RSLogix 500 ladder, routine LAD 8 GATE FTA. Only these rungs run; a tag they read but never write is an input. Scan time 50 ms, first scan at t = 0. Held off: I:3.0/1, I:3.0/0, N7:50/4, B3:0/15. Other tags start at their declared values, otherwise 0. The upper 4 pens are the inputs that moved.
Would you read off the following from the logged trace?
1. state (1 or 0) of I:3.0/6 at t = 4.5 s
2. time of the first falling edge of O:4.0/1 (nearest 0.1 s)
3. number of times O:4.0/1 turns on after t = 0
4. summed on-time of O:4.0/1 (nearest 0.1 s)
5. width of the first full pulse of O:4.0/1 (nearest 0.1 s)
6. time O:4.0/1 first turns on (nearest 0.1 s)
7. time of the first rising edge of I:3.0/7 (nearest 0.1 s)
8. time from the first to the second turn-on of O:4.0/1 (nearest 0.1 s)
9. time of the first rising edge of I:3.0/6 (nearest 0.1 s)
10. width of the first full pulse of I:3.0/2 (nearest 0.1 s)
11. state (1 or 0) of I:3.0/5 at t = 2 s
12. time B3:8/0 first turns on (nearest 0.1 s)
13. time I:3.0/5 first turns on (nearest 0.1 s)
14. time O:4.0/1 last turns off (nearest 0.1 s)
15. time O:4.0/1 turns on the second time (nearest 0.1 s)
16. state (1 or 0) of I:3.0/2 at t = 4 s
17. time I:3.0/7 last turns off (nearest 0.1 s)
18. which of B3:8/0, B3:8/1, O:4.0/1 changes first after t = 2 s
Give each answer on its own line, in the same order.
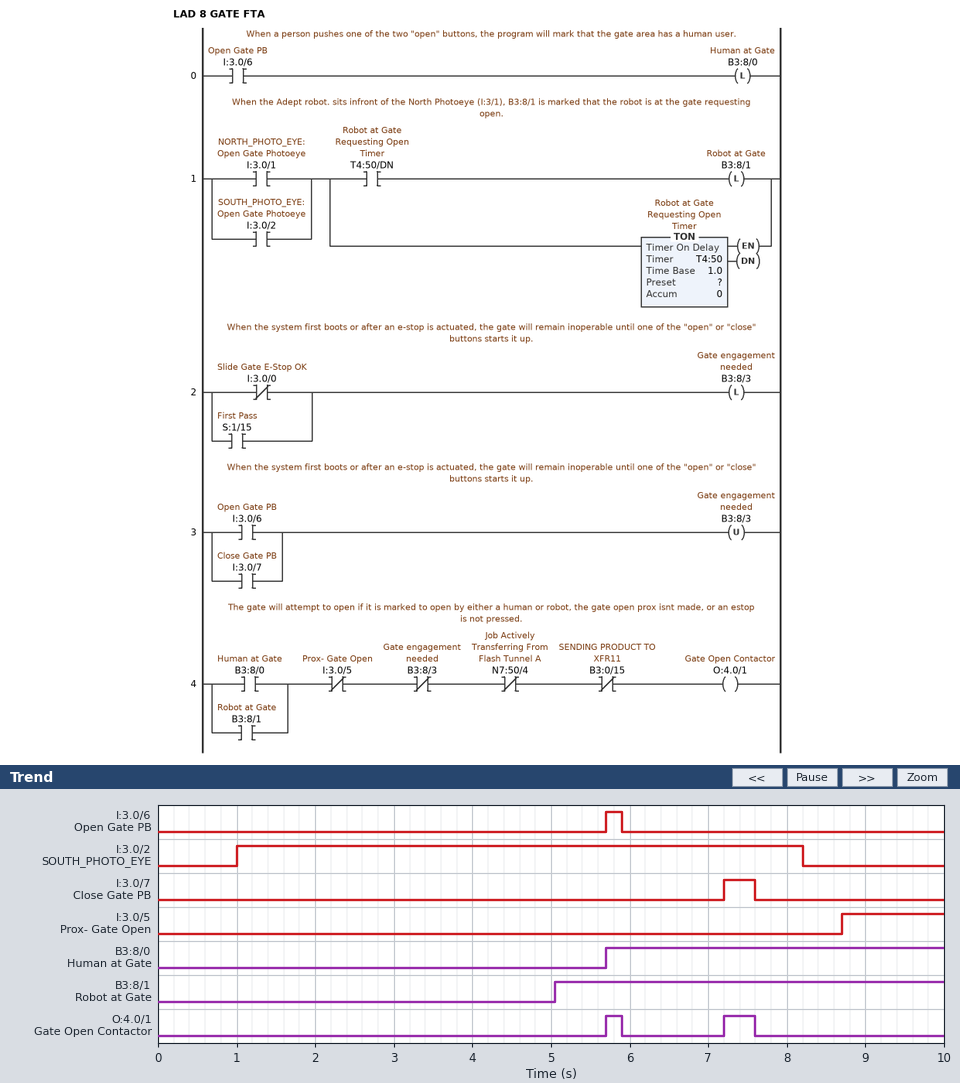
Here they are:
0
5.9 s
2
0.6 s
0.2 s
5.7 s
7.2 s
1.5 s
5.7 s
7.2 s
0
5.7 s
8.7 s
7.6 s
7.2 s
1
7.6 s
B3:8/1
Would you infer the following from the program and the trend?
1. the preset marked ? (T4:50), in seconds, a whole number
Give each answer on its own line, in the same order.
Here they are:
4 s
